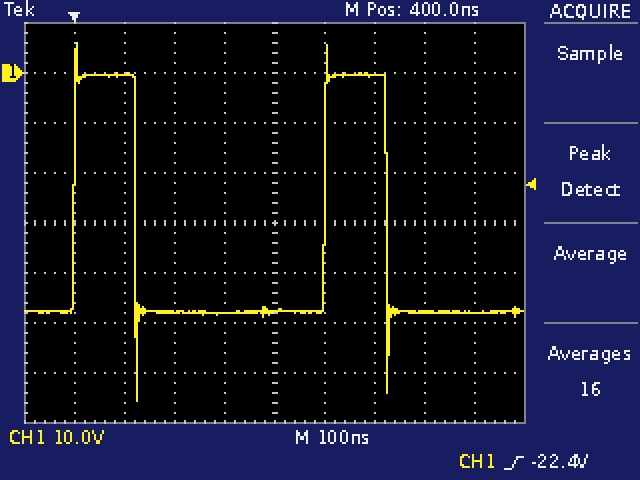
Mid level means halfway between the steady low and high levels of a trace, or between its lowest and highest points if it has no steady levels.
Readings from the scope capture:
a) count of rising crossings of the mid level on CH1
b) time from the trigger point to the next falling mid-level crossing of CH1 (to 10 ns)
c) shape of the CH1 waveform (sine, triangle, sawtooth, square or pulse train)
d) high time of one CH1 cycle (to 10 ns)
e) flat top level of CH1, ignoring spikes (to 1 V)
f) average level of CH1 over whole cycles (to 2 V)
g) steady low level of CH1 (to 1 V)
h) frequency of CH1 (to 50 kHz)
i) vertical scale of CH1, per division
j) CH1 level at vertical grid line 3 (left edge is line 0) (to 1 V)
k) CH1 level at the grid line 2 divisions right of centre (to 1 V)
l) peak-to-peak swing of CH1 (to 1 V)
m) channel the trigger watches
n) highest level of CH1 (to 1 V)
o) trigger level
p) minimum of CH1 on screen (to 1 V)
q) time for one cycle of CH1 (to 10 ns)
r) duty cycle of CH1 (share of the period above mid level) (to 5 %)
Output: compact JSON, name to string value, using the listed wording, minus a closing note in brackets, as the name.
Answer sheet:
{"count of rising crossings of the mid level on CH1": "2", "time from the trigger point to the next falling mid-level crossing of CH1": "120 ns", "shape of the CH1 waveform": "pulse train", "high time of one CH1 cycle": "120 ns", "flat top level of CH1, ignoring spikes": "0 V", "average level of CH1 over whole cycles": "-36 V", "steady low level of CH1": "-48 V", "frequency of CH1": "2.00 MHz", "vertical scale of CH1, per division": "10 V", "CH1 level at vertical grid line 3 (left edge is line 0)": "-48 V", "CH1 level at the grid line 2 divisions right of centre": "0 V", "peak-to-peak swing of CH1": "72 V", "channel the trigger watches": "CH1", "highest level of CH1": "6 V", "trigger level": "-22.4 V", "minimum of CH1 on screen": "-66 V", "time for one cycle of CH1": "500 ns", "duty cycle of CH1 (share of the period above mid level)": "25 %"}
